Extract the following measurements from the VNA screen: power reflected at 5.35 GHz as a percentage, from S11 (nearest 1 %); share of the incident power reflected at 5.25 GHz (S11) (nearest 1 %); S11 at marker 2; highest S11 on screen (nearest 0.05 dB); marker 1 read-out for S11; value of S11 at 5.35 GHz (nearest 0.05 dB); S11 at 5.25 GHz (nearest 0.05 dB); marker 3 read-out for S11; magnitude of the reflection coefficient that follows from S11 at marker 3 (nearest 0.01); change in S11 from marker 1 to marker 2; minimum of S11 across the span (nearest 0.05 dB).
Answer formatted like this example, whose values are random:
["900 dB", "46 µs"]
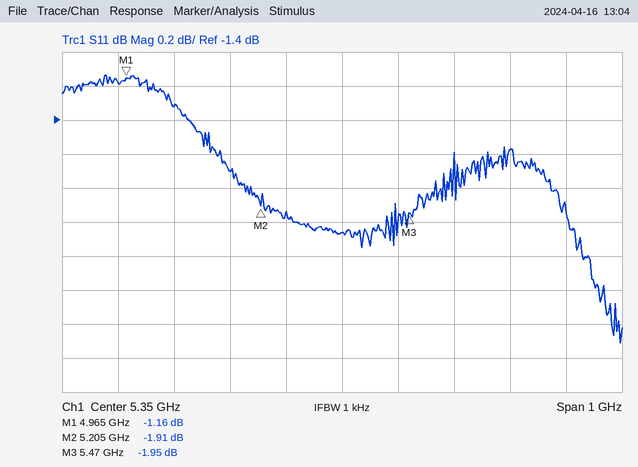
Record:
["62 %", "64 %", "-1.91 dB", "-1.15 dB", "-1.16 dB", "-2.05 dB", "-1.95 dB", "-1.95 dB", "0.80", "-0.75 dB", "-2.70 dB"]
